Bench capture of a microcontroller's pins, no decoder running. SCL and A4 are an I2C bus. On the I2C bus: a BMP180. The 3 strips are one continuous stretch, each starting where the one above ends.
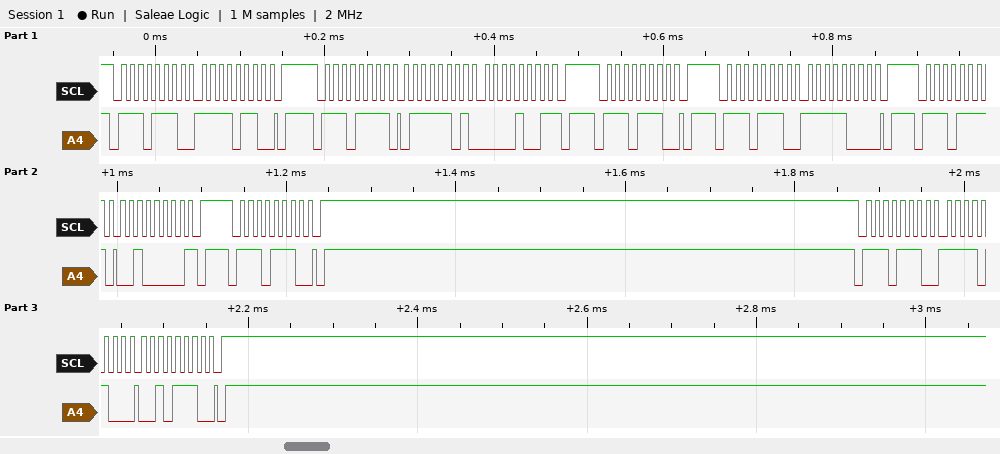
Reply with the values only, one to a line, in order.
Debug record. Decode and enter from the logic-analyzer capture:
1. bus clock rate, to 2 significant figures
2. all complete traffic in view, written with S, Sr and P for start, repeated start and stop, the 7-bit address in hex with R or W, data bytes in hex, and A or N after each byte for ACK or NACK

100 kHz
S 77W A F6 A P S 77R A 7D A 09 N P S 77W A P S 77W A F8 A P S 77R A 20 N P S 77W A P S 77W A F4 A 2E A P
